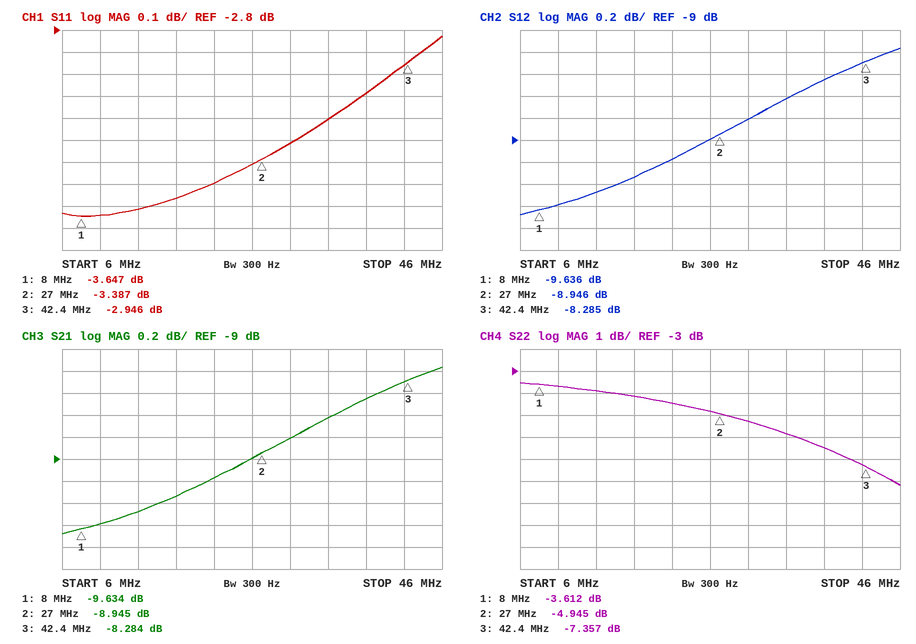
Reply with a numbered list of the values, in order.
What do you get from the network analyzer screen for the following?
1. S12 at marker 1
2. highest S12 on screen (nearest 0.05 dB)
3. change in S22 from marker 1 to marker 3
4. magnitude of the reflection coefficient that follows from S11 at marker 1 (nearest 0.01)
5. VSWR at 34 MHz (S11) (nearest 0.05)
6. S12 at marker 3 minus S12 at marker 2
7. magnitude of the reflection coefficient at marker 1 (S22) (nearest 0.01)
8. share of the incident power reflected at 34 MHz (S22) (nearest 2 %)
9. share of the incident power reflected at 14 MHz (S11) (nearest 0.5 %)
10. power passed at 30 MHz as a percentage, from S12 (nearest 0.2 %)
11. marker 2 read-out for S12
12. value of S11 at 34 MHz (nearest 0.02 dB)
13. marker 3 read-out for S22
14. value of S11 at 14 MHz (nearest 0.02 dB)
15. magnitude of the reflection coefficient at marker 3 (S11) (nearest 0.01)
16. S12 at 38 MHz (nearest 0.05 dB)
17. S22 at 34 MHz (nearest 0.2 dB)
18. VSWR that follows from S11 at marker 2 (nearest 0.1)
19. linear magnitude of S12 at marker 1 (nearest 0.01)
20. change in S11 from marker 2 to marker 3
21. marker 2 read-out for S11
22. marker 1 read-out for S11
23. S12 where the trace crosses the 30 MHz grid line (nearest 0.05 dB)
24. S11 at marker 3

1. -9.636 dB
2. -8.15 dB
3. -3.745 dB
4. 0.66
5. 5.50
6. 0.661 dB
7. 0.66
8. 26 %
9. 43.5 %
10. 13.2 %
11. -8.946 dB
12. -3.20 dB
13. -7.357 dB
14. -3.62 dB
15. 0.71
16. -8.45 dB
17. -5.8 dB
18. 5.2
19. 0.33
20. 0.441 dB
21. -3.387 dB
22. -3.647 dB
23. -8.80 dB
24. -2.946 dB
